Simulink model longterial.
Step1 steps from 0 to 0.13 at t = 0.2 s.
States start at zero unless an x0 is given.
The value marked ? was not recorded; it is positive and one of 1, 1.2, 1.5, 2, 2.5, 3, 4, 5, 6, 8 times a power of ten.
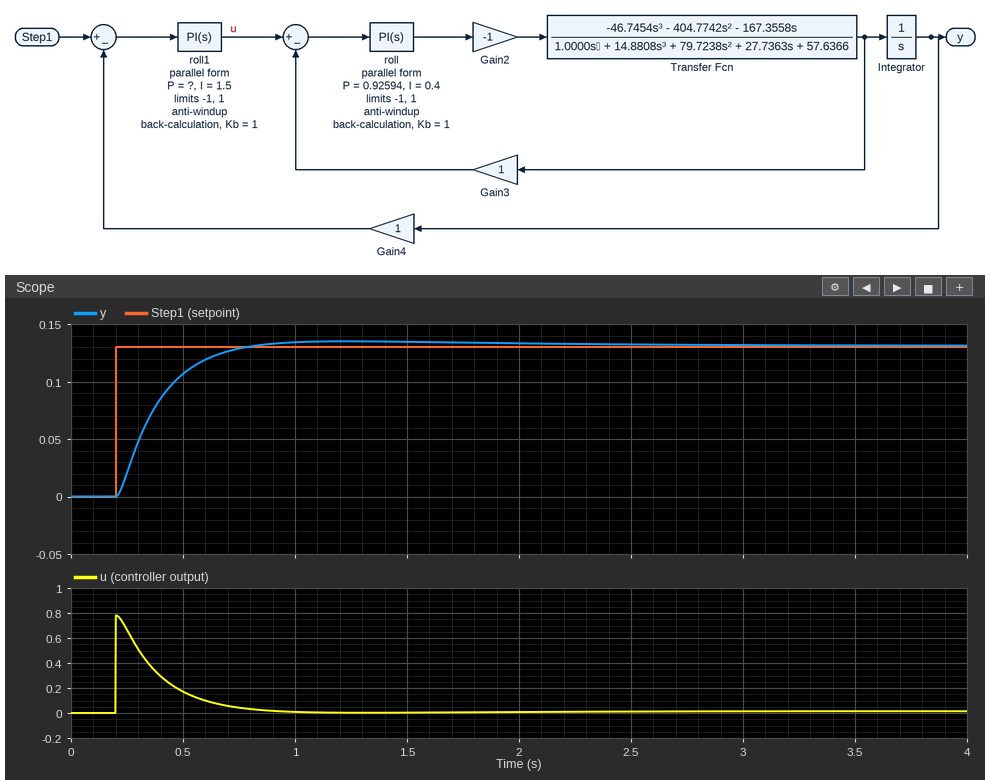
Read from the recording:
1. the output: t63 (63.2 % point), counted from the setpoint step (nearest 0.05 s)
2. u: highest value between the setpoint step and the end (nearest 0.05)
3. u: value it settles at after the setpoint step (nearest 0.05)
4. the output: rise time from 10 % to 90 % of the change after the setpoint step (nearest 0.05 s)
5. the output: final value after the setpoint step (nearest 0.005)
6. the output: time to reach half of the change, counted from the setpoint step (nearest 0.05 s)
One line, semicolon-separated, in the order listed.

0.20 s; 0.80; 0.00; 0.35 s; 0.130; 0.15 s
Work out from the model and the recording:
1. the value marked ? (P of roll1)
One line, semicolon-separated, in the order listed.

6
